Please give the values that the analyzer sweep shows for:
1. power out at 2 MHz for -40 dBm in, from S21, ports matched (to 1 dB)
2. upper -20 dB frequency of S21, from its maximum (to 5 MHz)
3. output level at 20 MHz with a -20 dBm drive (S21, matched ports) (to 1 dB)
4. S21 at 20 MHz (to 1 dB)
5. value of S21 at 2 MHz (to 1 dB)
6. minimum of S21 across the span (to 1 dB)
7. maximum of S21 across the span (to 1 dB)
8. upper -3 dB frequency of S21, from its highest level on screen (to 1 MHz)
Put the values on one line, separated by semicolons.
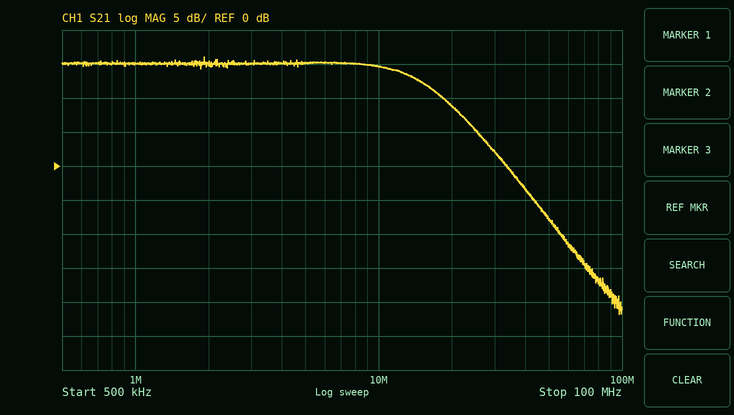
-25 dBm; 40 MHz; -11 dBm; 9 dB; 15 dB; -22 dB; 16 dB; 14 MHz
